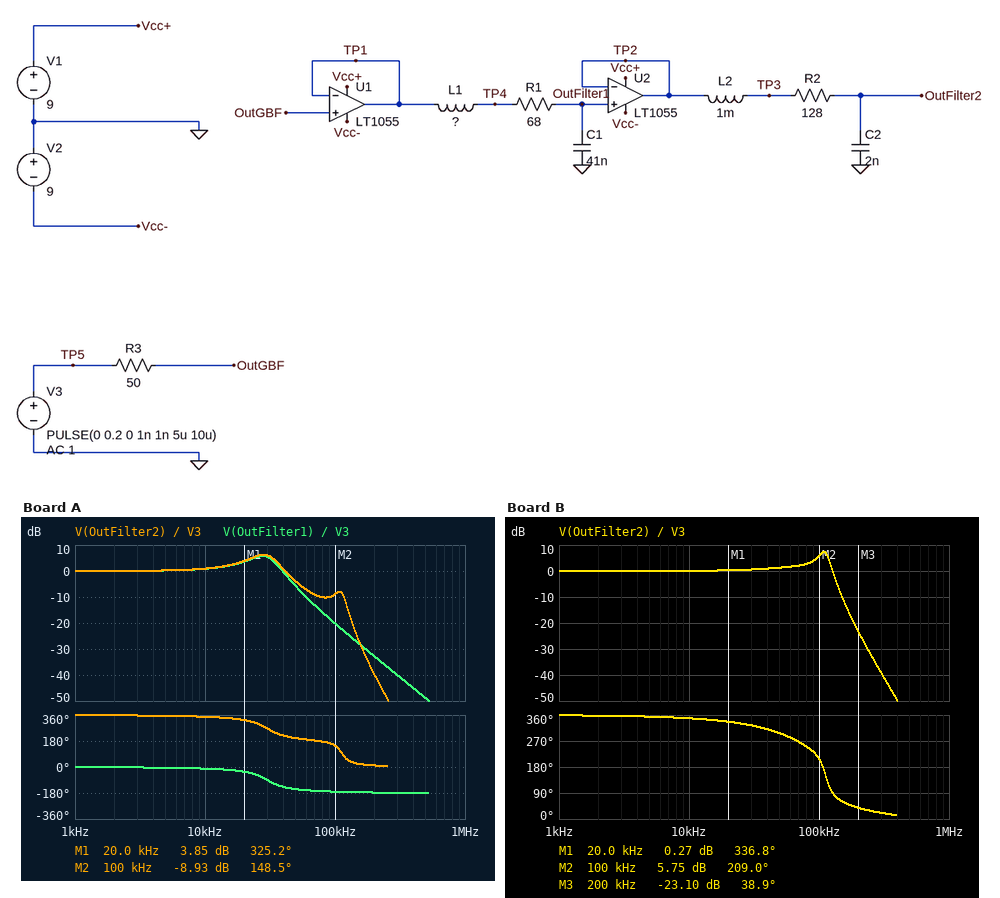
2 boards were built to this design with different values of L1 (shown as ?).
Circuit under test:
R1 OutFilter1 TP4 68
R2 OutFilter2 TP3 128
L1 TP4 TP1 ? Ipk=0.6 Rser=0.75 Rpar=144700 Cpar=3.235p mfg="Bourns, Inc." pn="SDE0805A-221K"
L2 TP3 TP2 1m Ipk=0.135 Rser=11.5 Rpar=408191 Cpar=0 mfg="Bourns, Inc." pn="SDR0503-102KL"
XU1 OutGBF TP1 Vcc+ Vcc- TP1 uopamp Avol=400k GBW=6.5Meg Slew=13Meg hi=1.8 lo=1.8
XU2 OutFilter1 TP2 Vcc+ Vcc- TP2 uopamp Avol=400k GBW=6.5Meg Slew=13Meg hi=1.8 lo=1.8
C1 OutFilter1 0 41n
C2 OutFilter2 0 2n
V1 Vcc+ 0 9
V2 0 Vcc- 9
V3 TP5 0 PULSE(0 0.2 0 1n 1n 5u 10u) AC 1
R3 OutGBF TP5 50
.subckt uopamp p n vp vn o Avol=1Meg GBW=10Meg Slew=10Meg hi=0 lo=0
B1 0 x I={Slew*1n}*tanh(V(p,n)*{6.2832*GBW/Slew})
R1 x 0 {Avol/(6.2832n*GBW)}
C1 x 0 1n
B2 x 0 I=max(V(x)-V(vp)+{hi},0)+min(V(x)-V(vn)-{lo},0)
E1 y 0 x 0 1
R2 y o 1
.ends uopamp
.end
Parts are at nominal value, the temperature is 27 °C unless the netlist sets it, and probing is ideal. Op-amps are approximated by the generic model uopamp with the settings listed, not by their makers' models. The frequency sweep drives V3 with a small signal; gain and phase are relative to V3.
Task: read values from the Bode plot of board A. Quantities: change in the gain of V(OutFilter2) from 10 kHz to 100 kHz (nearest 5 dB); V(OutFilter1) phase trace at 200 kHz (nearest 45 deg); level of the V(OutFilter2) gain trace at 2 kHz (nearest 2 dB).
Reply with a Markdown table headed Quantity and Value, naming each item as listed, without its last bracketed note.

| Quantity | Value |
|---|---|
| change in the gain of V(OutFilter2) from 10 kHz to 100 kHz | -10 dB |
| V(OutFilter1) phase trace at 200 kHz | -180 deg |
| level of the V(OutFilter2) gain trace at 2 kHz | 0 dB |
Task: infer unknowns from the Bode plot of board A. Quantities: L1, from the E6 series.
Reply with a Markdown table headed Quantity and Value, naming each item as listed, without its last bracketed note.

| Quantity | Value |
|---|---|
| L1, from the E6 series | 680 µH |
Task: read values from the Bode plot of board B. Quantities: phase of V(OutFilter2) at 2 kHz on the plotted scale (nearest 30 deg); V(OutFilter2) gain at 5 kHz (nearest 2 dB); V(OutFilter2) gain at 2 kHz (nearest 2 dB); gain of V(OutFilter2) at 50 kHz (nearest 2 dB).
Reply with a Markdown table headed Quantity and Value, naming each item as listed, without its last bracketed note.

| Quantity | Value |
|---|---|
| phase of V(OutFilter2) at 2 kHz on the plotted scale | 360 deg |
| V(OutFilter2) gain at 5 kHz | 0 dB |
| V(OutFilter2) gain at 2 kHz | 0 dB |
| gain of V(OutFilter2) at 50 kHz | 2 dB |
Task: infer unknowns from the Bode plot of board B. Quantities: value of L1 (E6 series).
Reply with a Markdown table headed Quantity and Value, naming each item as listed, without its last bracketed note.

| Quantity | Value |
|---|---|
| value of L1 | 100 µH |
